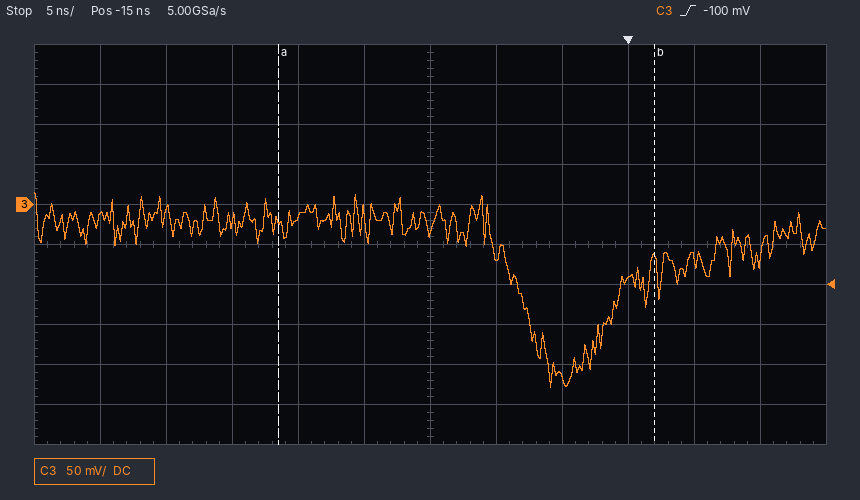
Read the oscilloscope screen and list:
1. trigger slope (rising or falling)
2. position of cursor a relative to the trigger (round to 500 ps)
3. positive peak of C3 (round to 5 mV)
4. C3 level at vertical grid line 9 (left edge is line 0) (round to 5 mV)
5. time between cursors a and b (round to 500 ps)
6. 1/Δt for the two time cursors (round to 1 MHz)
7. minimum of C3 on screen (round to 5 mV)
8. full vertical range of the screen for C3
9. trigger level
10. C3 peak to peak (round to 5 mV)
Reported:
rising
-26.5 ns
15 mV
-95 mV
28.5 ns
35 MHz
-230 mV
500 mV
-100 mV
245 mV
